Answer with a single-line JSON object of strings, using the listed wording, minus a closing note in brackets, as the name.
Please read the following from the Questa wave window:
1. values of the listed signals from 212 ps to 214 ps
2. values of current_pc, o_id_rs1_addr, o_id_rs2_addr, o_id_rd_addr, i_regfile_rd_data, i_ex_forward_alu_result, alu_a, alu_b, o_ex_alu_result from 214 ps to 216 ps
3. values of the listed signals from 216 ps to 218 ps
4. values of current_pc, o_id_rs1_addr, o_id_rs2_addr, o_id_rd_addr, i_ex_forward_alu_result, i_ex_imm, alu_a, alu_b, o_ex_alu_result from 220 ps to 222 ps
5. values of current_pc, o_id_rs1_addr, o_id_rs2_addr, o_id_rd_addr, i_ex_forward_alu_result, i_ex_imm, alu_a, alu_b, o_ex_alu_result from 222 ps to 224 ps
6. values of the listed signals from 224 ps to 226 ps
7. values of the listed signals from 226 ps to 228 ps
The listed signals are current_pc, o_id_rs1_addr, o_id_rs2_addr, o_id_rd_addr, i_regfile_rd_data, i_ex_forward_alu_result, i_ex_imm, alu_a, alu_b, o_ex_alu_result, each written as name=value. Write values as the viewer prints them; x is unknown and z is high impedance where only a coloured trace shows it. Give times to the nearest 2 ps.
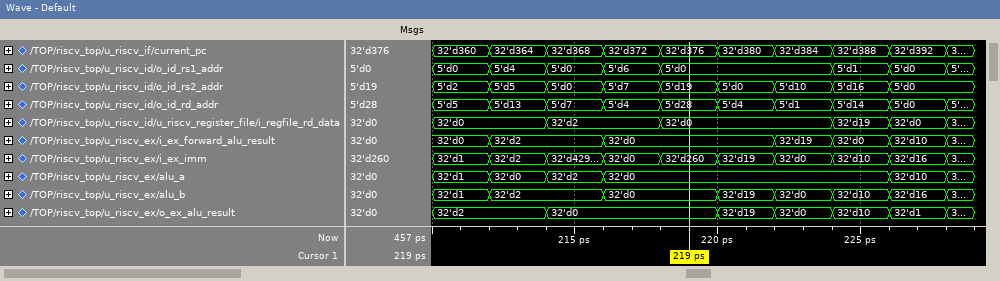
{"values of the listed signals from 212 ps to 214 ps": "current_pc=32'd364, o_id_rs1_addr=5'd4, o_id_rs2_addr=5'd5, o_id_rd_addr=5'd13, i_regfile_rd_data=32'd0, i_ex_forward_alu_result=32'd2, i_ex_imm=32'd2, alu_a=32'd0, alu_b=32'd2, o_ex_alu_result=32'd2", "values of current_pc, o_id_rs1_addr, o_id_rs2_addr, o_id_rd_addr, i_regfile_rd_data, i_ex_forward_alu_result, alu_a, alu_b, o_ex_alu_result from 214 ps to 216 ps": "current_pc=32'd368, o_id_rs1_addr=5'd0, o_id_rs2_addr=5'd0, o_id_rd_addr=5'd7, i_regfile_rd_data=32'd2, i_ex_forward_alu_result=32'd2, alu_a=32'd2, alu_b=32'd2, o_ex_alu_result=32'd0", "values of the listed signals from 216 ps to 218 ps": "current_pc=32'd372, o_id_rs1_addr=5'd6, o_id_rs2_addr=5'd7, o_id_rd_addr=5'd4, i_regfile_rd_data=32'd2, i_ex_forward_alu_result=32'd0, i_ex_imm=32'd0, alu_a=32'd0, alu_b=32'd0, o_ex_alu_result=32'd0", "values of current_pc, o_id_rs1_addr, o_id_rs2_addr, o_id_rd_addr, i_ex_forward_alu_result, i_ex_imm, alu_a, alu_b, o_ex_alu_result from 220 ps to 222 ps": "current_pc=32'd380, o_id_rs1_addr=5'd0, o_id_rs2_addr=5'd0, o_id_rd_addr=5'd4, i_ex_forward_alu_result=32'd0, i_ex_imm=32'd19, alu_a=32'd0, alu_b=32'd19, o_ex_alu_result=32'd19", "values of current_pc, o_id_rs1_addr, o_id_rs2_addr, o_id_rd_addr, i_ex_forward_alu_result, i_ex_imm, alu_a, alu_b, o_ex_alu_result from 222 ps to 224 ps": "current_pc=32'd384, o_id_rs1_addr=5'd0, o_id_rs2_addr=5'd10, o_id_rd_addr=5'd1, i_ex_forward_alu_result=32'd19, i_ex_imm=32'd0, alu_a=32'd0, alu_b=32'd0, o_ex_alu_result=32'd0", "values of the listed signals from 224 ps to 226 ps": "current_pc=32'd388, o_id_rs1_addr=5'd1, o_id_rs2_addr=5'd16, o_id_rd_addr=5'd14, i_regfile_rd_data=32'd19, i_ex_forward_alu_result=32'd0, i_ex_imm=32'd10, alu_a=32'd0, alu_b=32'd10, o_ex_alu_result=32'd10", "values of the listed signals from 226 ps to 228 ps": "current_pc=32'd392, o_id_rs1_addr=5'd0, o_id_rs2_addr=5'd0, o_id_rd_addr=5'd0, i_regfile_rd_data=32'd0, i_ex_forward_alu_result=32'd10, i_ex_imm=32'd16, alu_a=32'd10, alu_b=32'd16, o_ex_alu_result=32'd1"}
